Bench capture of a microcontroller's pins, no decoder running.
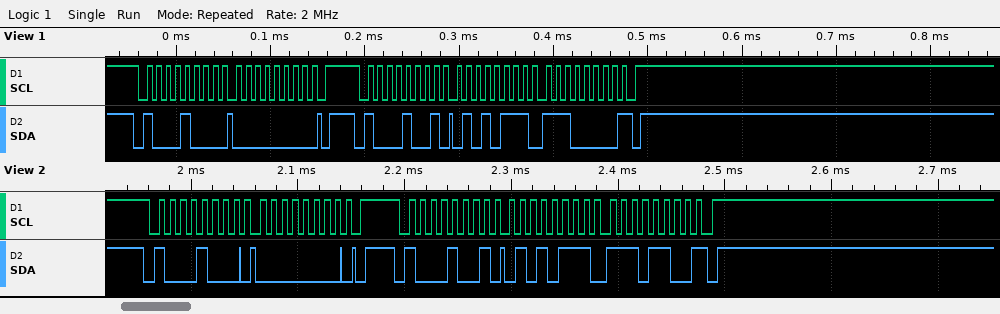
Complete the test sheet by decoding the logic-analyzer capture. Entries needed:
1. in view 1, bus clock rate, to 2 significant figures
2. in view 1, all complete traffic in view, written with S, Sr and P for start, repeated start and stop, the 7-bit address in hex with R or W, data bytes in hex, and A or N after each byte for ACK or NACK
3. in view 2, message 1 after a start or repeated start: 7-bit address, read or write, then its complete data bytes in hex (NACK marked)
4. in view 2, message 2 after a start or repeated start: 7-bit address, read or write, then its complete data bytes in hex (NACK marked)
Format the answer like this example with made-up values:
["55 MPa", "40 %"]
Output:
["100 kHz", "S 44W A 00 A P S 44R A 57 A E0 N P", "0x44 write: 00", "0x44 read: 57 EC NACK"]
